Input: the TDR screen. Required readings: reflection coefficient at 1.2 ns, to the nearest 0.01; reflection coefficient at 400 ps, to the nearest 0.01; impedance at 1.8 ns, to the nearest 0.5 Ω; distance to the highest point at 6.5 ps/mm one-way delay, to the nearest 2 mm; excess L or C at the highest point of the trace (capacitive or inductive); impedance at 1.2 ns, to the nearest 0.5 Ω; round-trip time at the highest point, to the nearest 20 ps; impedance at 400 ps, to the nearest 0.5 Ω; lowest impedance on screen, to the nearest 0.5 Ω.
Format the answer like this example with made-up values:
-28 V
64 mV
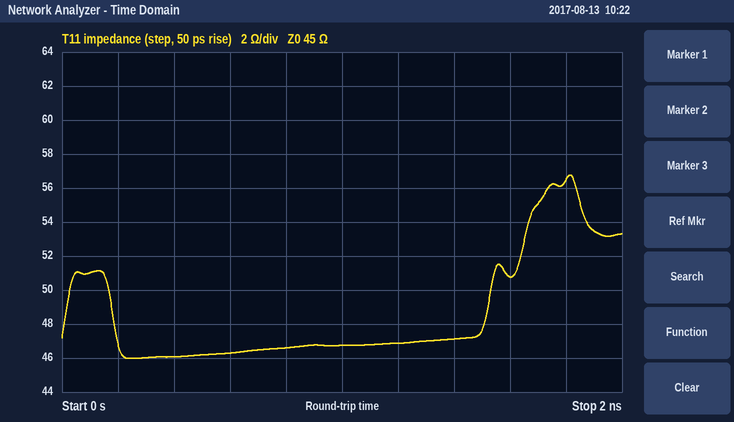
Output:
+0.02
+0.01
56.5 Ω
140 mm
inductive
47.0 Ω
1.82 ns
46.0 Ω
46.0 Ω
